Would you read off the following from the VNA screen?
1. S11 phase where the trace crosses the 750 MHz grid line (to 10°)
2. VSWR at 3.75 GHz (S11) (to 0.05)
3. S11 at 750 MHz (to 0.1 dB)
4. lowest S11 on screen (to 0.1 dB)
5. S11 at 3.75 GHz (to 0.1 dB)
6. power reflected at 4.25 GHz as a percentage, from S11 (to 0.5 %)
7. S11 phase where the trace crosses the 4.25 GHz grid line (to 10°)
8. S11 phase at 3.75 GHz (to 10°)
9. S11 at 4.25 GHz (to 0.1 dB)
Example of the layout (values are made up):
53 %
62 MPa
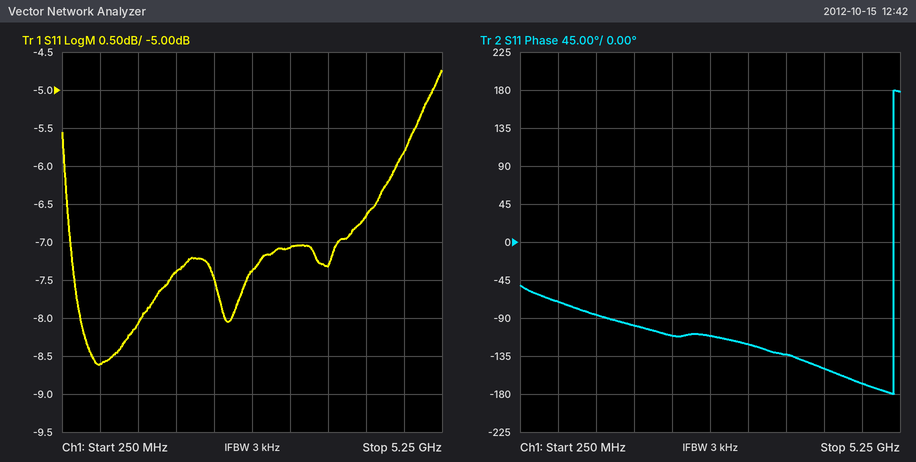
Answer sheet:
-70°
2.50
-8.6 dB
-8.6 dB
-7.3 dB
21.5 %
-150°
-130°
-6.7 dB
